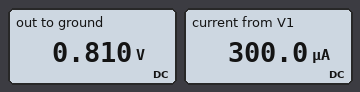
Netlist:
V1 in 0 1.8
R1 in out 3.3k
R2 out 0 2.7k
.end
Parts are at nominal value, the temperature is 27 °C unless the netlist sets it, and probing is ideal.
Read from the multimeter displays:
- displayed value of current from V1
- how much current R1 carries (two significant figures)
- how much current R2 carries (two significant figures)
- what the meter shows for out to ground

300.0 µA
300 µA
300 µA
0.810 V
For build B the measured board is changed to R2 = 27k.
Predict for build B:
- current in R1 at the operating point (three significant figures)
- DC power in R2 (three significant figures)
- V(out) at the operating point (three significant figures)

59.4 µA
95.3 µW
1.60 V
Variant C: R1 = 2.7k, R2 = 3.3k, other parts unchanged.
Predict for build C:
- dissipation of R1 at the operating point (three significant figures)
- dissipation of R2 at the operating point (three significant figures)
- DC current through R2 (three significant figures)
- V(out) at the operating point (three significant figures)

243 µW
297 µW
300 µA
990 mV
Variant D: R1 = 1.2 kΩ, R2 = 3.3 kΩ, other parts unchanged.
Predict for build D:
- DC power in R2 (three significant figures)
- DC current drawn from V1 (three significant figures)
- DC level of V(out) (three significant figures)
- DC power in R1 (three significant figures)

528 µW
400 µA
1.32 V
192 µW
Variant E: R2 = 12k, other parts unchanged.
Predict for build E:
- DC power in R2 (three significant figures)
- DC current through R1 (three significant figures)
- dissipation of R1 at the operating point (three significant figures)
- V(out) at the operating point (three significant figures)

166 µW
118 µA
45.7 µW
1.41 V
